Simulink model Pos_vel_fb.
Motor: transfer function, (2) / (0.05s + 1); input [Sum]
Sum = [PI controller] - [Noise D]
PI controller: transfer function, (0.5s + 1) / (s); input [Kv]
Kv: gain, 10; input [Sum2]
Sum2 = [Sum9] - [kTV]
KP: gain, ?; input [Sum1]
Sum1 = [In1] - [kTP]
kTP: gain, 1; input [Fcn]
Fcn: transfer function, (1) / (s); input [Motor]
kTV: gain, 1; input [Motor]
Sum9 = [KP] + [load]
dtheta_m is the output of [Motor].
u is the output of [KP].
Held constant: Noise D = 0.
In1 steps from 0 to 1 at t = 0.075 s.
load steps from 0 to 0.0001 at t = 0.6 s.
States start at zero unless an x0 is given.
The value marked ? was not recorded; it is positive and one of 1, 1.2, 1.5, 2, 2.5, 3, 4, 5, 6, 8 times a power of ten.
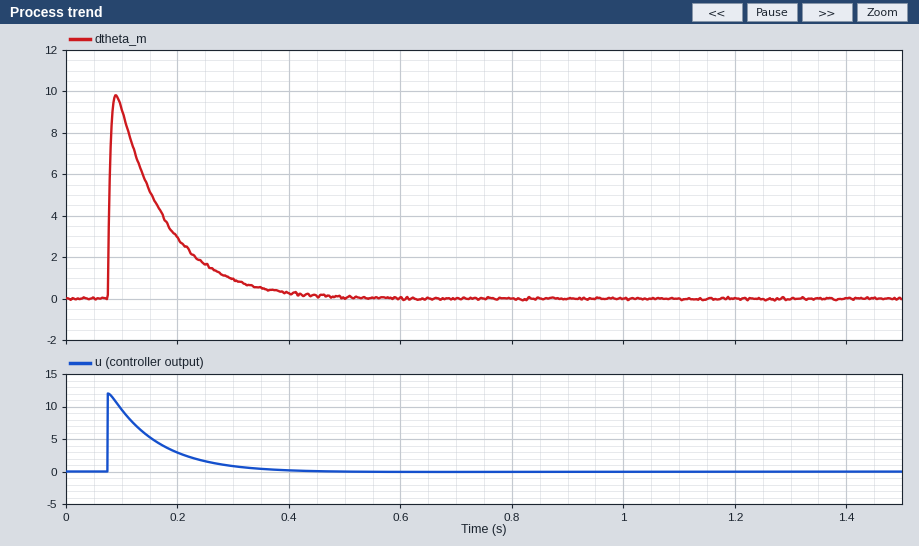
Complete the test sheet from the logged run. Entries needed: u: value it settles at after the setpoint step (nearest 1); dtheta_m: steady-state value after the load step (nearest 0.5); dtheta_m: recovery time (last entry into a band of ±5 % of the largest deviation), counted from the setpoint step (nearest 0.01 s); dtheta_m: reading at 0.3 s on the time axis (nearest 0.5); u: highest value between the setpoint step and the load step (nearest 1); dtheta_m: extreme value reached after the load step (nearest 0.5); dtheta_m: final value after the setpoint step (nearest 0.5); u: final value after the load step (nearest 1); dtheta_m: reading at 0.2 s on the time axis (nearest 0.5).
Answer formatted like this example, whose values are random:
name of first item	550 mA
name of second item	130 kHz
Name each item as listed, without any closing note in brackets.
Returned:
u: value it settles at after the setpoint step	0
dtheta_m: steady-state value after the load step	0.0
dtheta_m: recovery time (last entry into a band of ±5 % of the largest deviation), counted from the setpoint step	0.28 s
dtheta_m: reading at 0.3 s on the time axis	1.0
u: highest value between the setpoint step and the load step	12
dtheta_m: extreme value reached after the load step	0.0
dtheta_m: final value after the setpoint step	0.0
u: final value after the load step	0
dtheta_m: reading at 0.2 s on the time axis	3.0
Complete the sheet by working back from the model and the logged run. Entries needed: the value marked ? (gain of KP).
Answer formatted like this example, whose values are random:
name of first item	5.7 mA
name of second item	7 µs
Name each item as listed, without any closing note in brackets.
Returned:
the value marked ?	12
